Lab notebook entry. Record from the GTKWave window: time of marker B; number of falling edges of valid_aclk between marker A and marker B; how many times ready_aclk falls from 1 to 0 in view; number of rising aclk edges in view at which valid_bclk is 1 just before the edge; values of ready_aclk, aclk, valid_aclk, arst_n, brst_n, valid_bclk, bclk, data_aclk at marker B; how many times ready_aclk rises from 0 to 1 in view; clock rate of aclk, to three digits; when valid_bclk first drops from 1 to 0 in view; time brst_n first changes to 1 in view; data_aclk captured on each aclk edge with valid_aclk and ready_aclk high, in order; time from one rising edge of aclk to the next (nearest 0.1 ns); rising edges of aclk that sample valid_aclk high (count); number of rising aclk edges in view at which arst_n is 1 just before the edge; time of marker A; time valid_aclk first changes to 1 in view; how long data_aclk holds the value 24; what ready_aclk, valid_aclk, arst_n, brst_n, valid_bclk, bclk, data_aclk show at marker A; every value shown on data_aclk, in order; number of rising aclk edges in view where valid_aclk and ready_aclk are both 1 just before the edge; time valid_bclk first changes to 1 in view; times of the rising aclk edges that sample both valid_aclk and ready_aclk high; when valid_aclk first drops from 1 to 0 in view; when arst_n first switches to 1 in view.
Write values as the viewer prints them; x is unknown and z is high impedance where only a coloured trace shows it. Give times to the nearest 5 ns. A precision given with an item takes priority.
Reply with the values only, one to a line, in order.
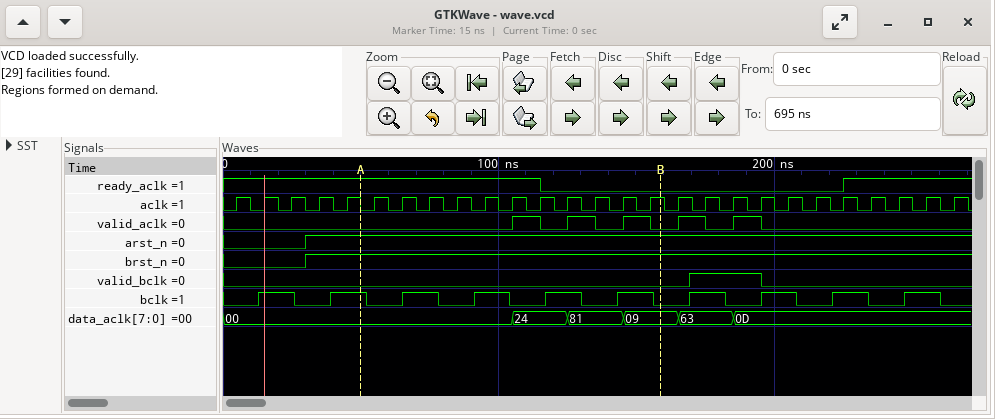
160 ns
3
1
3
ready_aclk=0, aclk=1, valid_aclk=0, arst_n=1, brst_n=1, valid_bclk=0, bclk=0, data_aclk=09
1
100 MHz
195 ns
30 ns
24
10 ns
5
24
50 ns
105 ns
20 ns
ready_aclk=1, valid_aclk=0, arst_n=1, brst_n=1, valid_bclk=0, bclk=1, data_aclk=00
00, 24, 81, 09, 63, 0D
1
170 ns
115 ns
115 ns
30 ns
